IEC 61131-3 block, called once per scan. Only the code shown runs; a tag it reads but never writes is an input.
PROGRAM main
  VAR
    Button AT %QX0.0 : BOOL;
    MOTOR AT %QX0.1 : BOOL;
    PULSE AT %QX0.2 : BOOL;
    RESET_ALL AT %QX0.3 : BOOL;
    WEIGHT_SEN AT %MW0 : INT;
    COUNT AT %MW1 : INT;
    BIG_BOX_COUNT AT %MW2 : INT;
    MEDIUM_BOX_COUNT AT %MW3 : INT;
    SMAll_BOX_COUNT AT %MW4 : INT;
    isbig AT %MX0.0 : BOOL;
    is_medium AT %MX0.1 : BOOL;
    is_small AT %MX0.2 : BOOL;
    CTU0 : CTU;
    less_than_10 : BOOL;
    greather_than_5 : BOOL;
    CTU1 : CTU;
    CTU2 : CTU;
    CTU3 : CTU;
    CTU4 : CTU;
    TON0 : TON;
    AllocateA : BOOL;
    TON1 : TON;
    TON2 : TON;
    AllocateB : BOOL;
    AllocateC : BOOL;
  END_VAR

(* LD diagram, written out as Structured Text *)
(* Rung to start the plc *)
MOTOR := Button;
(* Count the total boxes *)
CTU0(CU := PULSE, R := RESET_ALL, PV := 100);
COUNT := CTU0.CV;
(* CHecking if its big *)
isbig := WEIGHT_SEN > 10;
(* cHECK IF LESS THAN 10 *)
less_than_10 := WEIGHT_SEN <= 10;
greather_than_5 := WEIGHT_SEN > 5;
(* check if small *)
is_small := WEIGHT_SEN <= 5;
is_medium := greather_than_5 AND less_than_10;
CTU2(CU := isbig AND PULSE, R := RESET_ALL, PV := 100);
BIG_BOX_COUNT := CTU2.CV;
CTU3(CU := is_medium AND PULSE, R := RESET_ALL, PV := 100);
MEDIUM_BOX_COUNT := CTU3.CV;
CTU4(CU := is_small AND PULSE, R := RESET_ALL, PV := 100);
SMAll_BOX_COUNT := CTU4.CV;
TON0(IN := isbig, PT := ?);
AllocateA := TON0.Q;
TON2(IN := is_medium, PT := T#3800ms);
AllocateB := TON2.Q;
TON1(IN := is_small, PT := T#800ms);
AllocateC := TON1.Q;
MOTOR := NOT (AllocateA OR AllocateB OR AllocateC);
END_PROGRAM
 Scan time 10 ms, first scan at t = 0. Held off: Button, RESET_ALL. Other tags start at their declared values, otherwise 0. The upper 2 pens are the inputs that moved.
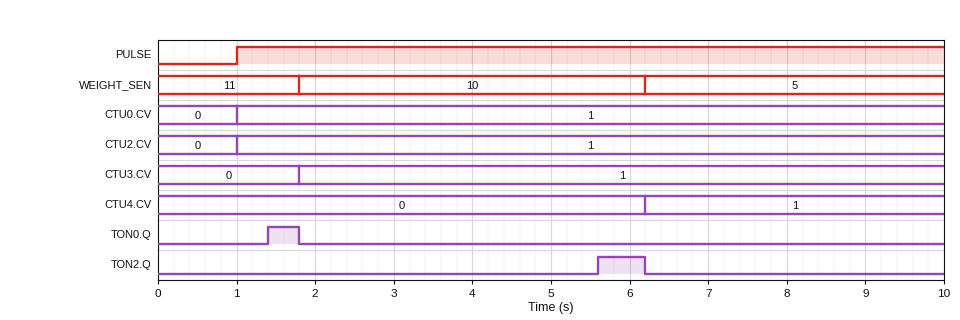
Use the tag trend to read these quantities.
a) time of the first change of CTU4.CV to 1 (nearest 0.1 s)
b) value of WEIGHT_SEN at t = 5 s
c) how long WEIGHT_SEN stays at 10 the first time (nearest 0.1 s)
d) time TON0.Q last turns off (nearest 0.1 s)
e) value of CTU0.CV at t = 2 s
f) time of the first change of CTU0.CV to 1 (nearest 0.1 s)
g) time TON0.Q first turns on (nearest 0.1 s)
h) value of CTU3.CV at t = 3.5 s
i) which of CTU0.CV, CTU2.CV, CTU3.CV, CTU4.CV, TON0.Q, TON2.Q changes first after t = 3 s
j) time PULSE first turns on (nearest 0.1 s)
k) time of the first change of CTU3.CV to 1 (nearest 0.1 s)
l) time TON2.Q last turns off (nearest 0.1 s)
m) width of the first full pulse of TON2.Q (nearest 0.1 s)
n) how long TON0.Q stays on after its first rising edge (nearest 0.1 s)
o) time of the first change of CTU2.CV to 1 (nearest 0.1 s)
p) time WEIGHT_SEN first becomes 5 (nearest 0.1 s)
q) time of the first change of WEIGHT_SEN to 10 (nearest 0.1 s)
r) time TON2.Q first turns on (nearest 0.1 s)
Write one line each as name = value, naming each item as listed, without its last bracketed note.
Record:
time of the first change of CTU4.CV to 1 = 6.2 s
value of WEIGHT_SEN at t = 5 s = 10
how long WEIGHT_SEN stays at 10 the first time = 4.4 s
time TON0.Q last turns off = 1.8 s
value of CTU0.CV at t = 2 s = 1
time of the first change of CTU0.CV to 1 = 1.0 s
time TON0.Q first turns on = 1.4 s
value of CTU3.CV at t = 3.5 s = 1
which of CTU0.CV, CTU2.CV, CTU3.CV, CTU4.CV, TON0.Q, TON2.Q changes first after t = 3 s = TON2.Q
time PULSE first turns on = 1.0 s
time of the first change of CTU3.CV to 1 = 1.8 s
time TON2.Q last turns off = 6.2 s
width of the first full pulse of TON2.Q = 0.6 s
how long TON0.Q stays on after its first rising edge = 0.4 s
time of the first change of CTU2.CV to 1 = 1.0 s
time WEIGHT_SEN first becomes 5 = 6.2 s
time of the first change of WEIGHT_SEN to 10 = 1.8 s
time TON2.Q first turns on = 5.6 s
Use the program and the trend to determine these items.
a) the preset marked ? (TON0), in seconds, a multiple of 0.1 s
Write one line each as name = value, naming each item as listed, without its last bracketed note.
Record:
the preset marked ? (TON0), in seconds, a multiple of 0.1 s = 1.4 s
